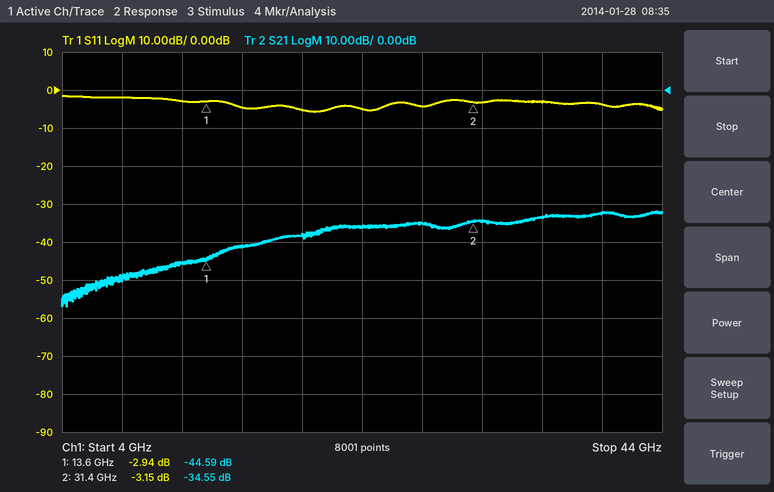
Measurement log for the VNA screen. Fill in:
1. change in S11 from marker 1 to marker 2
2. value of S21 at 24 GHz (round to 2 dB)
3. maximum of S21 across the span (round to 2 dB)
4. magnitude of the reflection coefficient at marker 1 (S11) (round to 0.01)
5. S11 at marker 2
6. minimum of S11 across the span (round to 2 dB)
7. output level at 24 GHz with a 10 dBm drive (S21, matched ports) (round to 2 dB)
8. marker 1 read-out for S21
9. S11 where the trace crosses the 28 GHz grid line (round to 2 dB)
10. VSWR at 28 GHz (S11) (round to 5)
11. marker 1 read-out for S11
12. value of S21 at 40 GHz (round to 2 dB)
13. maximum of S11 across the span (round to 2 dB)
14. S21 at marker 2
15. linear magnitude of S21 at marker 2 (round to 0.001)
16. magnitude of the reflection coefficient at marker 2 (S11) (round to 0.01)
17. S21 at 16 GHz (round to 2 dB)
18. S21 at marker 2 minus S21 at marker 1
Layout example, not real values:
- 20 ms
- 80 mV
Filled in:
- -0.21 dB
- -36 dB
- -32 dB
- 0.71
- -3.15 dB
- -6 dB
- -26 dBm
- -44.59 dB
- -4 dB
- 5
- -2.94 dB
- -32 dB
- -2 dB
- -34.55 dB
- 0.019
- 0.70
- -42 dB
- 10.04 dB
